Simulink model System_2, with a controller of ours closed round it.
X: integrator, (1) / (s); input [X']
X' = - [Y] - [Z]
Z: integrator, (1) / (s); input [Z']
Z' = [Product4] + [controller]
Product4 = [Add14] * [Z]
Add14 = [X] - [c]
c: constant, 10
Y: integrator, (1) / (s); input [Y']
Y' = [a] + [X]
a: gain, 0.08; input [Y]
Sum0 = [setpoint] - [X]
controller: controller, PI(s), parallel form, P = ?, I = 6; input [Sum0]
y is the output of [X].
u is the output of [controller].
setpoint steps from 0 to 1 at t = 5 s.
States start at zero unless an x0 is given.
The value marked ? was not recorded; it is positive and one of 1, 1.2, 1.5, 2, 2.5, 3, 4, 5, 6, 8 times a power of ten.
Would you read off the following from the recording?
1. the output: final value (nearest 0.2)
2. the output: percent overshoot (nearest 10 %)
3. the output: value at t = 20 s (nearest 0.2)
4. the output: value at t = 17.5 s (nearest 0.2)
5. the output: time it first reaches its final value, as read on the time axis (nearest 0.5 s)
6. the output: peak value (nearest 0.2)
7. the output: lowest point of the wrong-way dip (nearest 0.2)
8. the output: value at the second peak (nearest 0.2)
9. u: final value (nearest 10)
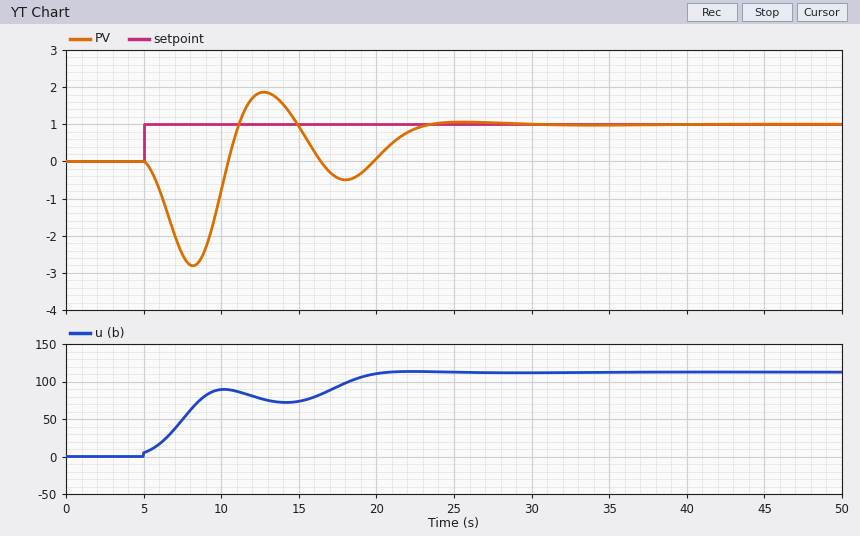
1.0
90 %
0.0
-0.4
11.0 s
1.8
-2.8
1.0
110
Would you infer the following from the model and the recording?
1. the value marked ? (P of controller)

5
